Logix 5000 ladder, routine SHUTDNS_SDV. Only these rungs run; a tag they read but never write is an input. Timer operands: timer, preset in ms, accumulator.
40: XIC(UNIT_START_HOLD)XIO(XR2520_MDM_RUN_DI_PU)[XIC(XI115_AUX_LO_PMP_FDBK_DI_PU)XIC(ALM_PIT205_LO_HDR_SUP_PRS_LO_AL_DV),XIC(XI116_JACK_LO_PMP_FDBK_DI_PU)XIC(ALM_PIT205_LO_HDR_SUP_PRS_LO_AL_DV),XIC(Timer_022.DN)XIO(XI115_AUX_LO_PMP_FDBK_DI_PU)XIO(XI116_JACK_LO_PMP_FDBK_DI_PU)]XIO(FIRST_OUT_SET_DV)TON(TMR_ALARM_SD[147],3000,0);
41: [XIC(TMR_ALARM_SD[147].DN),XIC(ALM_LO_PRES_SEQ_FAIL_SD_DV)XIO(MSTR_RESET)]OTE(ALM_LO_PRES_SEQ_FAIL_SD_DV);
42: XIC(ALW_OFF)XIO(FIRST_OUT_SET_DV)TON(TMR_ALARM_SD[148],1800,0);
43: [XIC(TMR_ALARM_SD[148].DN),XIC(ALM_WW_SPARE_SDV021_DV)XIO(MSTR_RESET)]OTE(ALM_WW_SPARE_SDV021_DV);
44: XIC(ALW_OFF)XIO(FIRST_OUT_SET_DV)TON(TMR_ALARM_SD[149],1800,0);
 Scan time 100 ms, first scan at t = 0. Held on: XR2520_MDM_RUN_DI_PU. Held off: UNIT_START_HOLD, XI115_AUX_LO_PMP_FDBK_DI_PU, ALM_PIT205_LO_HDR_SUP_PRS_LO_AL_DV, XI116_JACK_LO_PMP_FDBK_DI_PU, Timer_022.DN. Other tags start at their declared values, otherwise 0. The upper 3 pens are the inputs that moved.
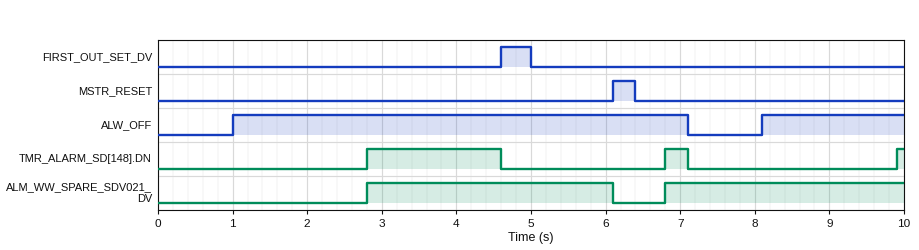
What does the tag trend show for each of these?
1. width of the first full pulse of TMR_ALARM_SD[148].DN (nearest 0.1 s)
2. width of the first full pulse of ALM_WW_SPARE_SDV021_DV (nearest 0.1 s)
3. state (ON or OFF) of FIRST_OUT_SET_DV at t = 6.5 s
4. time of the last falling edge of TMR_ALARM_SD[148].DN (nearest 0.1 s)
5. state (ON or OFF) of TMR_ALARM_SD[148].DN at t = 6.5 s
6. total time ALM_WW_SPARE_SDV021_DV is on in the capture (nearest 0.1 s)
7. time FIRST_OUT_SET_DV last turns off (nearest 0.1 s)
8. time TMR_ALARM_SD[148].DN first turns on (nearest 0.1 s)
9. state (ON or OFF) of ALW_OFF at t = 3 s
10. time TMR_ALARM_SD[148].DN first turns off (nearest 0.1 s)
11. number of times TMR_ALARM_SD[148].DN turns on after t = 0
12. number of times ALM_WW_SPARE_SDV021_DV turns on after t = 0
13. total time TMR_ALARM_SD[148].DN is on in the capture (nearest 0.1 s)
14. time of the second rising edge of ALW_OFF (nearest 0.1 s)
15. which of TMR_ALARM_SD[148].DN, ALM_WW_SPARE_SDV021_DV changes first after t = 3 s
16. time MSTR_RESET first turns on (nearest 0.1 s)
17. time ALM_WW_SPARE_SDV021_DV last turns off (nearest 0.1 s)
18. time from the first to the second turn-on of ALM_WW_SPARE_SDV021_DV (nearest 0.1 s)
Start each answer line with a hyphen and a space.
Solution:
- 1.8 s
- 3.3 s
- OFF
- 7.1 s
- OFF
- 6.5 s
- 5.0 s
- 2.8 s
- ON
- 4.6 s
- 3
- 2
- 2.2 s
- 8.1 s
- TMR_ALARM_SD[148].DN
- 6.1 s
- 6.1 s
- 4.0 s
